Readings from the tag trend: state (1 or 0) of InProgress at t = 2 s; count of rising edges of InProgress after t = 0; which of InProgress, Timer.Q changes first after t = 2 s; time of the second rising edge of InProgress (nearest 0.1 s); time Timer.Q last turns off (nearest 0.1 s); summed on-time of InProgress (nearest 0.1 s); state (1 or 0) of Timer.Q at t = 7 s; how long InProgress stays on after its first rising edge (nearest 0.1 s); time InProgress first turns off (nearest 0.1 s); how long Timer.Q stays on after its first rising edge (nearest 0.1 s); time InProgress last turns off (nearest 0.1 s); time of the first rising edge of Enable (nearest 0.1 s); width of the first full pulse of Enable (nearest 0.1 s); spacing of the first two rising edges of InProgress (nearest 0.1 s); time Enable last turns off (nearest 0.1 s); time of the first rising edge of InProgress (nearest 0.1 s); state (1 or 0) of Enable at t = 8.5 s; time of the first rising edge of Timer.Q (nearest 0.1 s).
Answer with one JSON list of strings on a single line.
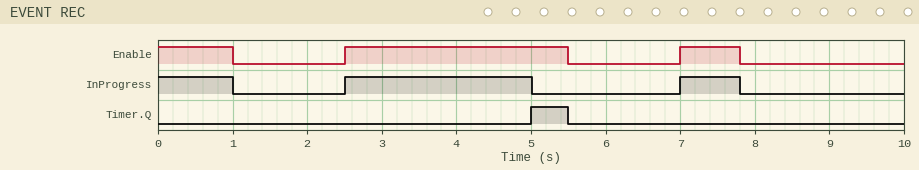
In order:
["0", "2", "InProgress", "7.0 s", "5.5 s", "4.3 s", "0", "2.5 s", "1.0 s", "0.5 s", "7.8 s", "2.5 s", "3.0 s", "4.5 s", "7.8 s", "2.5 s", "0", "5.0 s"]
